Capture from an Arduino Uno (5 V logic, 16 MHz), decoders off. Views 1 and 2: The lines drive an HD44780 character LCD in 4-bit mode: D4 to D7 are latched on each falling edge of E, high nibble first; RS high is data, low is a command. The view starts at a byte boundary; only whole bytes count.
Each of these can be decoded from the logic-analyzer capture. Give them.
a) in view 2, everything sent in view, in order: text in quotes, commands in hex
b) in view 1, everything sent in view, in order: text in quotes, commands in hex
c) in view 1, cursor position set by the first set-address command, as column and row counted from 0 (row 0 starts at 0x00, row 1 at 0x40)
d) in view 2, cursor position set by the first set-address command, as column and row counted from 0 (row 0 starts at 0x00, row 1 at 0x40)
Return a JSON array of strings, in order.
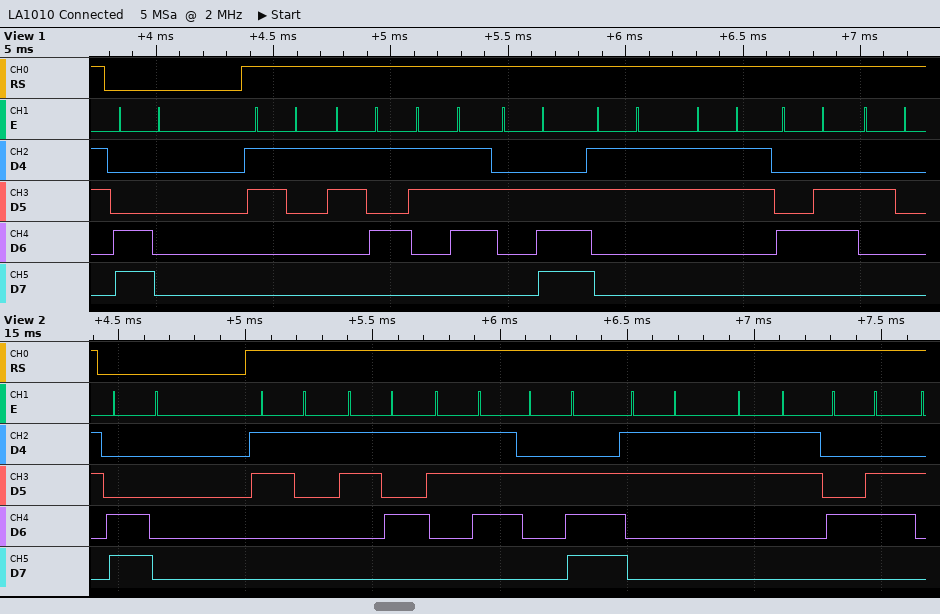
["0xC0 \"157.33F\"", "0xC0 \"157.33F \"", "column 0, row 1", "column 0, row 1"]
